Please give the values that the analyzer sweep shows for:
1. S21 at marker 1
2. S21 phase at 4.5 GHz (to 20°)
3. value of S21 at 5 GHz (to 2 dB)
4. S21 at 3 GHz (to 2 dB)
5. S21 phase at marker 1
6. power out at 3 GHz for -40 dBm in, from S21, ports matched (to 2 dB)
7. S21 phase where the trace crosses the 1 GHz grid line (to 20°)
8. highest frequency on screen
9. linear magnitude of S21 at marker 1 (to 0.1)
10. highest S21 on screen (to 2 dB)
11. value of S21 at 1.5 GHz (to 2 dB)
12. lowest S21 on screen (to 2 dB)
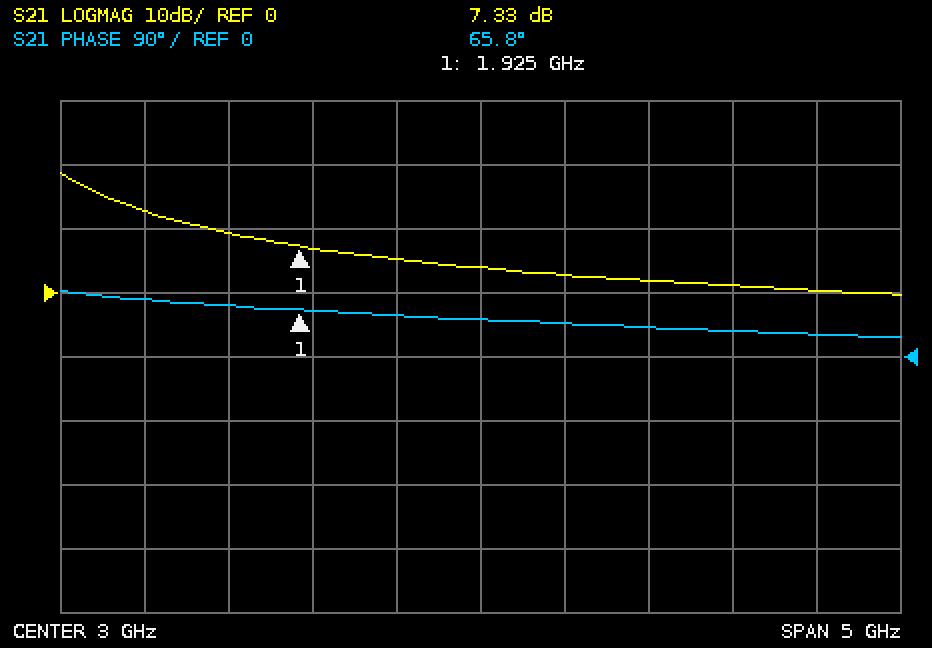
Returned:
7.33 dB
40°
0 dB
4 dB
65.8°
-36 dBm
80°
5.5 GHz
2.3
18 dB
10 dB
0 dB
